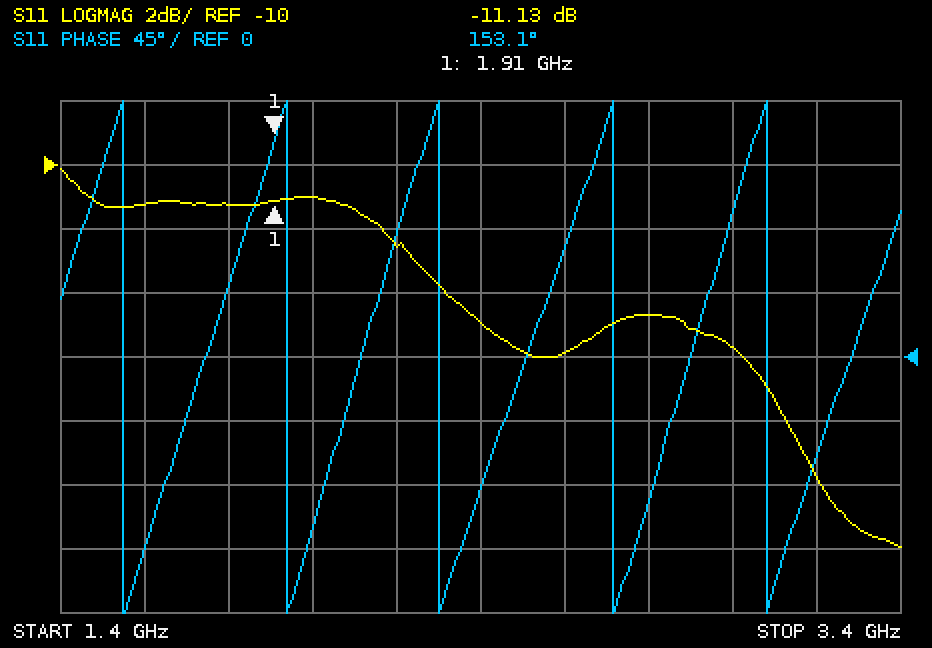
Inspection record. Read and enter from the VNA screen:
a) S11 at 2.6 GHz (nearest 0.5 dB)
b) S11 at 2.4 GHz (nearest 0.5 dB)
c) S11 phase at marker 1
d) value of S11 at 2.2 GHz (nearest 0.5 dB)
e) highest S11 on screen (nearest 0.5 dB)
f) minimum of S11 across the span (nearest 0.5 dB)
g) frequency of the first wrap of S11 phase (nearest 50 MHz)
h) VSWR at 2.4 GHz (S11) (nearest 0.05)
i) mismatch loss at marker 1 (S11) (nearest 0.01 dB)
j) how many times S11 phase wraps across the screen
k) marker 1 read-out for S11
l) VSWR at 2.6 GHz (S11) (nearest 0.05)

-16.0 dB
-15.0 dB
153.1°
-12.5 dB
-10.0 dB
-22.0 dB
1.55 GHz
1.45
0.35 dB
5
-11.13 dB
1.40
